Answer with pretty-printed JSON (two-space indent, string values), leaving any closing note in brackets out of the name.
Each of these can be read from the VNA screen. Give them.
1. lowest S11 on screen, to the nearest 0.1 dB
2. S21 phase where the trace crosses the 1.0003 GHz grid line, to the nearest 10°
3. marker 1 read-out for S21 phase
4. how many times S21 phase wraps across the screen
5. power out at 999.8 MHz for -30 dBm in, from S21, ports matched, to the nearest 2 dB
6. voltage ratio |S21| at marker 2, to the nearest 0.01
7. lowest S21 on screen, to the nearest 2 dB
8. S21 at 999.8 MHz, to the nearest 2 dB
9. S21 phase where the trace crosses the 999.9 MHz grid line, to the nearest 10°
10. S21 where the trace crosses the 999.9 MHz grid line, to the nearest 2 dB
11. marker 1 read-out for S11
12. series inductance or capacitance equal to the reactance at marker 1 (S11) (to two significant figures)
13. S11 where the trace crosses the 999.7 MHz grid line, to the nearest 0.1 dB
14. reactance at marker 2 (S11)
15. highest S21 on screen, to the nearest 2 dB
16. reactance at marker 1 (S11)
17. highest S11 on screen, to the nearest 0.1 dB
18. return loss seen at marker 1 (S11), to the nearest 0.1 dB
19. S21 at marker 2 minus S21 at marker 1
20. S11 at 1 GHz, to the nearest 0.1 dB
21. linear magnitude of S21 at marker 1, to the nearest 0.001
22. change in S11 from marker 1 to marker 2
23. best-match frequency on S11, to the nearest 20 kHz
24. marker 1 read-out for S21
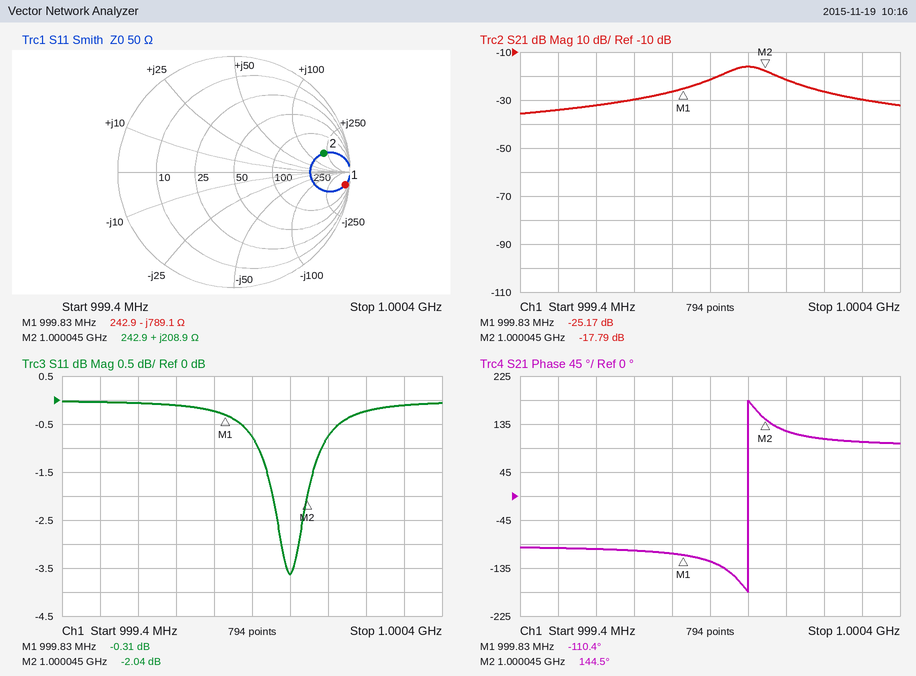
{
  "lowest S11 on screen, to the nearest 0.1 dB": "-3.6 dB",
  "S21 phase where the trace crosses the 1.0003 GHz grid line, to the nearest 10°": "100°",
  "marker 1 read-out for S21 phase": "-110.4°",
  "how many times S21 phase wraps across the screen": "1",
  "power out at 999.8 MHz for -30 dBm in, from S21, ports matched, to the nearest 2 dB": "-56 dBm",
  "voltage ratio |S21| at marker 2, to the nearest 0.01": "0.13",
  "lowest S21 on screen, to the nearest 2 dB": "-36 dB",
  "S21 at 999.8 MHz, to the nearest 2 dB": "-26 dB",
  "S21 phase where the trace crosses the 999.9 MHz grid line, to the nearest 10°": "-120°",
  "S21 where the trace crosses the 999.9 MHz grid line, to the nearest 2 dB": "-22 dB",
  "marker 1 read-out for S11": "-0.31 dB",
  "series inductance or capacitance equal to the reactance at marker 1 (S11)": "200 fF",
  "S11 where the trace crosses the 999.7 MHz grid line, to the nearest 0.1 dB": "-0.1 dB",
  "reactance at marker 2": "+208.9 Ω",
  "highest S21 on screen, to the nearest 2 dB": "-16 dB",
  "reactance at marker 1": "-789.1 Ω",
  "highest S11 on screen, to the nearest 0.1 dB": "0.0 dB",
  "return loss seen at marker 1 (S11), to the nearest 0.1 dB": "0.3 dB",
  "S21 at marker 2 minus S21 at marker 1": "7.38 dB",
  "S11 at 1 GHz, to the nearest 0.1 dB": "-3.6 dB",
  "linear magnitude of S21 at marker 1, to the nearest 0.001": "0.055",
  "change in S11 from marker 1 to marker 2": "-1.73 dB",
  "best-match frequency on S11, to the nearest 20 kHz": "1.00000 GHz",
  "marker 1 read-out for S21": "-25.17 dB"
}
